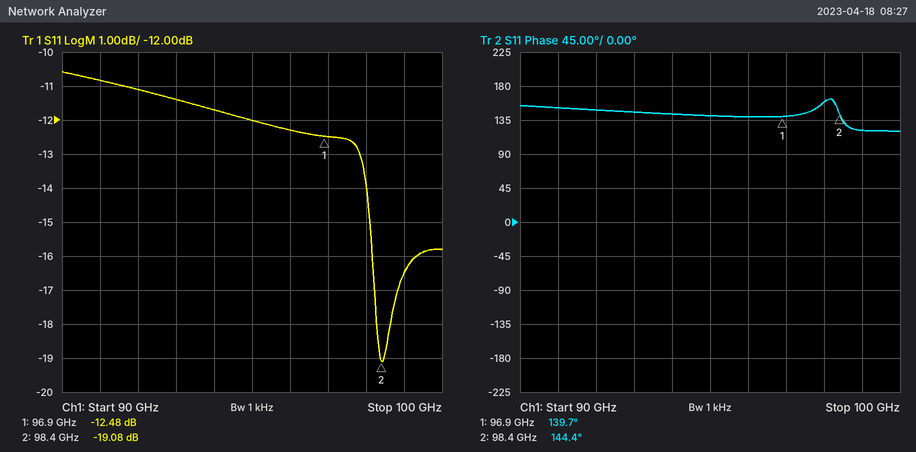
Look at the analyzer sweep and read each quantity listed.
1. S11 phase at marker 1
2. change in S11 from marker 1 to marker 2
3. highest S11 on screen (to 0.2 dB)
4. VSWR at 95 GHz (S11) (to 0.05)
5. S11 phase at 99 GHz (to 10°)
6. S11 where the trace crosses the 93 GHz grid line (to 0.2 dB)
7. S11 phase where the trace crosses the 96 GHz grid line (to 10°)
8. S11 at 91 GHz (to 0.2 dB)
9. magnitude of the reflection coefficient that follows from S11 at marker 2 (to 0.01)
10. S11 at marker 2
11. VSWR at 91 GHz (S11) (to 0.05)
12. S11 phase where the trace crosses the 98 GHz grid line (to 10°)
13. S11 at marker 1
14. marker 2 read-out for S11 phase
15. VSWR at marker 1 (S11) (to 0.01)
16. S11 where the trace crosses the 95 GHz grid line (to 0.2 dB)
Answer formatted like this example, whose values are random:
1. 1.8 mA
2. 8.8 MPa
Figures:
1. 139.7°
2. -6.60 dB
3. -10.6 dB
4. 1.65
5. 120°
6. -11.4 dB
7. 140°
8. -10.8 dB
9. 0.11
10. -19.08 dB
11. 1.80
12. 160°
13. -12.48 dB
14. 144.4°
15. 1.62
16. -12.0 dB
